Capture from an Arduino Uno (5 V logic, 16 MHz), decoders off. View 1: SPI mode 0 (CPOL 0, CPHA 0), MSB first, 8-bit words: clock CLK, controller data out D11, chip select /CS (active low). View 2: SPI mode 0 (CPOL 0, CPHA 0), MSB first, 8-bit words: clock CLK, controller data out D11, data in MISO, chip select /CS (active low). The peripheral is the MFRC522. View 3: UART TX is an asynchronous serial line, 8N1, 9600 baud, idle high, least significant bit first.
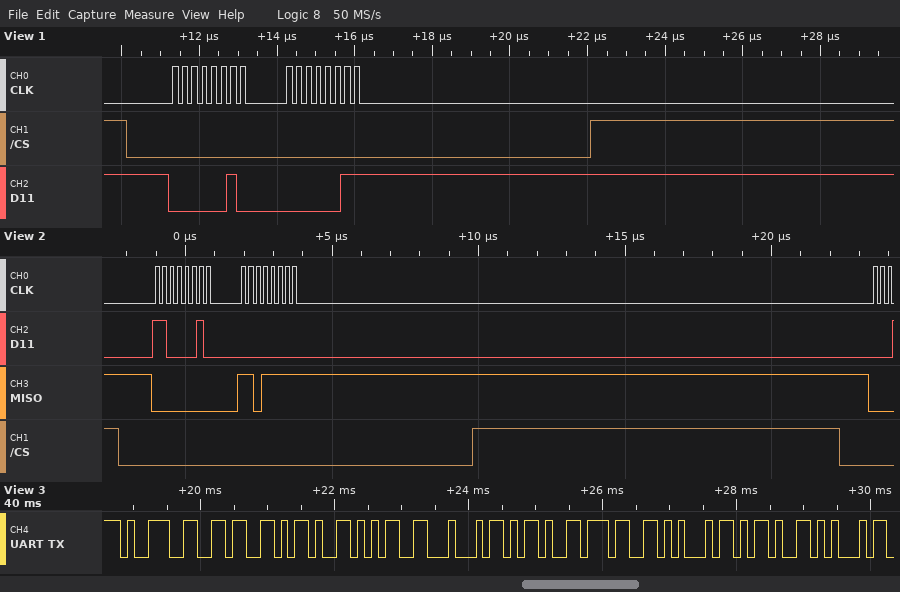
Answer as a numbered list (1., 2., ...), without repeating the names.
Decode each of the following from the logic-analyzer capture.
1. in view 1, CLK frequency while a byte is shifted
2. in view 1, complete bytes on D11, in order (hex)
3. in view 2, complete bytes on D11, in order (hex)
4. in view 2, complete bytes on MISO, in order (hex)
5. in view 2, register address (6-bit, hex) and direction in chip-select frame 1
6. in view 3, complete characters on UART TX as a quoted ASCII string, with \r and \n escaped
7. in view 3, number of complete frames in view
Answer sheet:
1. 4 MHz
2. 02 03
3. C2 00
4. 00 DF
5. 0x21 read
6. "96-5D-7E-E"
7. 10
